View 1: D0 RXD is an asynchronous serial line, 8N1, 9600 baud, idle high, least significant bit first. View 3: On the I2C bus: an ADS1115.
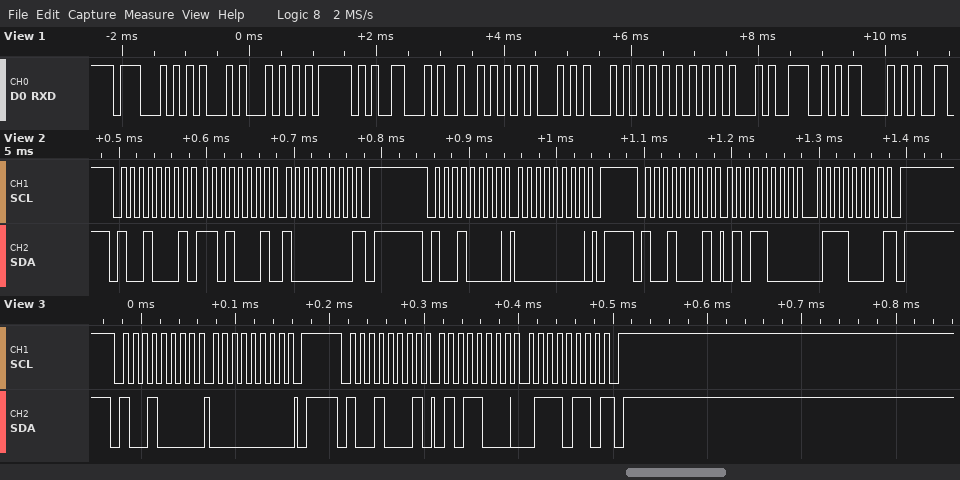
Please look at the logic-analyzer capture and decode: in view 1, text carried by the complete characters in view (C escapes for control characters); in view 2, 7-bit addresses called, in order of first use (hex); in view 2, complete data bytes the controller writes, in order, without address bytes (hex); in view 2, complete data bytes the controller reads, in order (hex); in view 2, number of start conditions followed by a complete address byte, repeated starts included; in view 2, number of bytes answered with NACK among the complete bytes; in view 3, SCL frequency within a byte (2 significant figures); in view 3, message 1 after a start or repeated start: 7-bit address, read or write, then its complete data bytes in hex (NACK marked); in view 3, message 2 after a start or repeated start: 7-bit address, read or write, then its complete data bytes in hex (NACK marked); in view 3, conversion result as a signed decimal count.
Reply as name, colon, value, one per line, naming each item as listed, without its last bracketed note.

in view 1, text carried by the complete characters in view: "GET_FREQUENC"
in view 2, 7-bit addresses called, in order of first use: 0x48
in view 2, complete data bytes the controller writes, in order, without address bytes: 00
in view 2, complete data bytes the controller reads, in order: D1 80 58 70
in view 2, number of start conditions followed by a complete address byte, repeated starts included: 3
in view 2, number of bytes answered with NACK among the complete bytes: 2
in view 3, SCL frequency within a byte: 100 kHz
in view 3, message 1 after a start or repeated start: 7-bit address, read or write, then its complete data bytes in hex: 0x48 write: 00
in view 3, message 2 after a start or repeated start: 7-bit address, read or write, then its complete data bytes in hex: 0x48 read: 58 76 NACK
in view 3, conversion result as a signed decimal count: 22646
